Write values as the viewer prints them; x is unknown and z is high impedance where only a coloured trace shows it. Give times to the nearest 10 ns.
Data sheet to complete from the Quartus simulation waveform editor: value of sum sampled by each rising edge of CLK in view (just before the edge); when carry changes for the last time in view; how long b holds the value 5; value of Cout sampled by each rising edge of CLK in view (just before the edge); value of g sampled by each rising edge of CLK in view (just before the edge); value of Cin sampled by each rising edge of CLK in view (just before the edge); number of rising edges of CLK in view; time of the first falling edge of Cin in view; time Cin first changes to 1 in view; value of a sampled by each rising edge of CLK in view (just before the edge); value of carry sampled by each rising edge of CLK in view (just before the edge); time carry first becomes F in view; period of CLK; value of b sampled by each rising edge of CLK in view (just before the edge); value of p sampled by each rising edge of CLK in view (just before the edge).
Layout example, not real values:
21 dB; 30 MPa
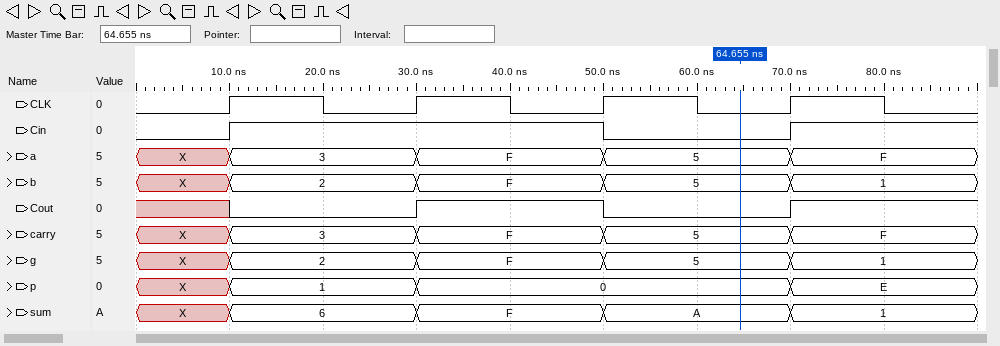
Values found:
X, 6, F, A; 70 ns; 20 ns; x 0 1 0; X, 2, F, 5; 0 1 1 0; 4; 50 ns; 10 ns; X, 3, F, 5; X, 3, F, 5; 30 ns; 20 ns; X, 2, F, 5; X, 1, 0, 0
